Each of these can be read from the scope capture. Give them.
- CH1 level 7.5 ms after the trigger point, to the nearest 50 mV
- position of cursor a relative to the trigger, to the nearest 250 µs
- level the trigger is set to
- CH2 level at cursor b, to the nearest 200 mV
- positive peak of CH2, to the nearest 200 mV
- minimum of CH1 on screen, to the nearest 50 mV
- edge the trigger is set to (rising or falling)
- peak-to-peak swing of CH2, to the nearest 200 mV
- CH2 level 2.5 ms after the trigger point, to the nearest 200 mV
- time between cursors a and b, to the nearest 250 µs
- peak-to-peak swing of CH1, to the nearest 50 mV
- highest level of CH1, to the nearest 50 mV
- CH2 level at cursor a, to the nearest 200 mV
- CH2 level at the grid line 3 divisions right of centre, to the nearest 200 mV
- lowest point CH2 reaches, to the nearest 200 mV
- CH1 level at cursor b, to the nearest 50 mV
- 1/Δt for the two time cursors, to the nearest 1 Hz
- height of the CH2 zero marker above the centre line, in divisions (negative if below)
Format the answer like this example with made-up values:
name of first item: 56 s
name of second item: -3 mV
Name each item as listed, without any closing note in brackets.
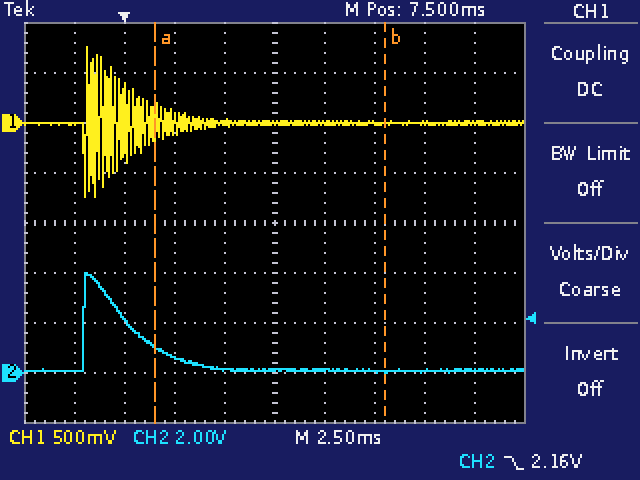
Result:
CH1 level 7.5 ms after the trigger point, to the nearest 50 mV: 0 mV
position of cursor a relative to the trigger, to the nearest 250 µs: +1.50 ms
level the trigger is set to: 2.16 V
CH2 level at cursor b, to the nearest 200 mV: 0.0 V
positive peak of CH2, to the nearest 200 mV: 4.0 V
minimum of CH1 on screen, to the nearest 50 mV: -750 mV
edge the trigger is set to: falling
peak-to-peak swing of CH2, to the nearest 200 mV: 4.0 V
CH2 level 2.5 ms after the trigger point, to the nearest 200 mV: 600 mV
time between cursors a and b, to the nearest 250 µs: 11.50 ms
peak-to-peak swing of CH1, to the nearest 50 mV: 1.50 V
highest level of CH1, to the nearest 50 mV: 750 mV
CH2 level at cursor a, to the nearest 200 mV: 1.0 V
CH2 level at the grid line 3 divisions right of centre, to the nearest 200 mV: 0.0 V
lowest point CH2 reaches, to the nearest 200 mV: 0.0 V
CH1 level at cursor b, to the nearest 50 mV: 0 mV
1/Δt for the two time cursors, to the nearest 1 Hz: 87 Hz
height of the CH2 zero marker above the centre line, in divisions: -3.0 div
